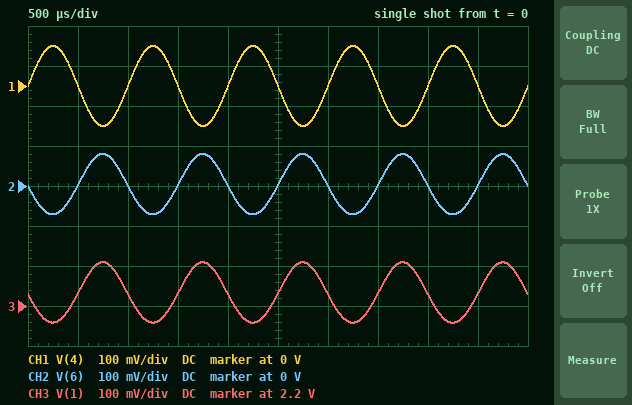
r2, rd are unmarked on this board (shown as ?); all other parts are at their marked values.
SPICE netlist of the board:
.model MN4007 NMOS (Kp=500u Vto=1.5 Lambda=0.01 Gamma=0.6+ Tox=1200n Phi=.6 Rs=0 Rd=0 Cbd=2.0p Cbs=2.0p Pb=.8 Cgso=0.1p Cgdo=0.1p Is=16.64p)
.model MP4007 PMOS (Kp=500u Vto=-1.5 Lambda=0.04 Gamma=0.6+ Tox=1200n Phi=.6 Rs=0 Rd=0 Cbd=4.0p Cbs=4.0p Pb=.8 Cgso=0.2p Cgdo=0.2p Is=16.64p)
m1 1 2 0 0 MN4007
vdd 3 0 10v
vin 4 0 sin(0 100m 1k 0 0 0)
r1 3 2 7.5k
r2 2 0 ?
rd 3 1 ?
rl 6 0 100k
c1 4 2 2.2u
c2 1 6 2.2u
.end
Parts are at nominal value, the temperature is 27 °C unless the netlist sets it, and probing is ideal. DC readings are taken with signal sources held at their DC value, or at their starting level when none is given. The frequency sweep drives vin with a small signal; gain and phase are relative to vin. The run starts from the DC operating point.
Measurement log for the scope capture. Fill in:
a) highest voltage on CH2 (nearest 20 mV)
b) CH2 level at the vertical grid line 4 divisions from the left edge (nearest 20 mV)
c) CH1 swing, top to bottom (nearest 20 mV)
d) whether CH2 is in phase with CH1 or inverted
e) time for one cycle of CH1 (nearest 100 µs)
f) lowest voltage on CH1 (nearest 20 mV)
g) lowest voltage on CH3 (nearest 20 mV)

80 mV
0 V
200 mV
inverted
1.0 ms
-100 mV
2.16 V
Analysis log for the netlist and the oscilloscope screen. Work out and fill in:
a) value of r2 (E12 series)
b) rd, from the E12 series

10 kΩ
2.2 kΩ
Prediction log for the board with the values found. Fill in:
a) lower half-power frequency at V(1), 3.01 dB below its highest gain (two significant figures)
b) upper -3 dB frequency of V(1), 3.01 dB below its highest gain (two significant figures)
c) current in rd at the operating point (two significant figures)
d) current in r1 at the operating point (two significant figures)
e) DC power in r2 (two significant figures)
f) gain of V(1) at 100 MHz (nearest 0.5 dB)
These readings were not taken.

17 Hz
220 MHz
3.5 mA
570 µA
3.3 mW
-3.5 dB
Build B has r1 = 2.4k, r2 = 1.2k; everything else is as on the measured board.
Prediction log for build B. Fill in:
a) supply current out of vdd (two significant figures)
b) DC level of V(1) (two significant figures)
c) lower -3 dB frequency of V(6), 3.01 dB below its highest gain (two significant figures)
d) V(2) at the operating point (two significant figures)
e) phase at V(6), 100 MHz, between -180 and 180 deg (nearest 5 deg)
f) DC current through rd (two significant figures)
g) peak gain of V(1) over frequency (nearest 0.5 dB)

3.7 mA
8.0 V
90 Hz
3.3 V
140 deg
910 µA
6.5 dB
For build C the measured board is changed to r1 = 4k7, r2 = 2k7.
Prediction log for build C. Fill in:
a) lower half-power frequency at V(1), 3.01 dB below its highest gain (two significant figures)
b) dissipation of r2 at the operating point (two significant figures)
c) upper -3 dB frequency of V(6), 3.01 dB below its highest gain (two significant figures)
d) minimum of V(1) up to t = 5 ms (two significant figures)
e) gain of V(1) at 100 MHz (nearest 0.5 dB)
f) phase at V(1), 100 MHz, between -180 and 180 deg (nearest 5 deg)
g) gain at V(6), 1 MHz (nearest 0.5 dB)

42 Hz
4.9 mW
120 MHz
7.0 V
5.5 dB
140 deg
7.5 dB
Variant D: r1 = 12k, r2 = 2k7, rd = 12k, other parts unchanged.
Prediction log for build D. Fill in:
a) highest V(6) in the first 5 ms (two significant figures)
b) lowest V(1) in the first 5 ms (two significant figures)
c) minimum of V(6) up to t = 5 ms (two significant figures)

170 mV
9.4 V
-220 mV
